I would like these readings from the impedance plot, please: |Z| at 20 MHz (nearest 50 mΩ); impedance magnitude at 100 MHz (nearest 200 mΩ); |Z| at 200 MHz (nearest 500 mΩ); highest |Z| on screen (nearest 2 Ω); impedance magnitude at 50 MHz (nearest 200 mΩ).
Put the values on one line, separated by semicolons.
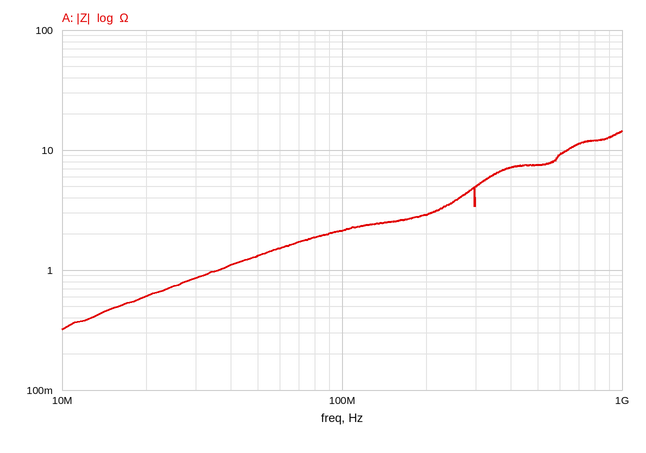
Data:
600 mΩ; 2.2 Ω; 3.0 Ω; 14 Ω; 1.4 Ω
